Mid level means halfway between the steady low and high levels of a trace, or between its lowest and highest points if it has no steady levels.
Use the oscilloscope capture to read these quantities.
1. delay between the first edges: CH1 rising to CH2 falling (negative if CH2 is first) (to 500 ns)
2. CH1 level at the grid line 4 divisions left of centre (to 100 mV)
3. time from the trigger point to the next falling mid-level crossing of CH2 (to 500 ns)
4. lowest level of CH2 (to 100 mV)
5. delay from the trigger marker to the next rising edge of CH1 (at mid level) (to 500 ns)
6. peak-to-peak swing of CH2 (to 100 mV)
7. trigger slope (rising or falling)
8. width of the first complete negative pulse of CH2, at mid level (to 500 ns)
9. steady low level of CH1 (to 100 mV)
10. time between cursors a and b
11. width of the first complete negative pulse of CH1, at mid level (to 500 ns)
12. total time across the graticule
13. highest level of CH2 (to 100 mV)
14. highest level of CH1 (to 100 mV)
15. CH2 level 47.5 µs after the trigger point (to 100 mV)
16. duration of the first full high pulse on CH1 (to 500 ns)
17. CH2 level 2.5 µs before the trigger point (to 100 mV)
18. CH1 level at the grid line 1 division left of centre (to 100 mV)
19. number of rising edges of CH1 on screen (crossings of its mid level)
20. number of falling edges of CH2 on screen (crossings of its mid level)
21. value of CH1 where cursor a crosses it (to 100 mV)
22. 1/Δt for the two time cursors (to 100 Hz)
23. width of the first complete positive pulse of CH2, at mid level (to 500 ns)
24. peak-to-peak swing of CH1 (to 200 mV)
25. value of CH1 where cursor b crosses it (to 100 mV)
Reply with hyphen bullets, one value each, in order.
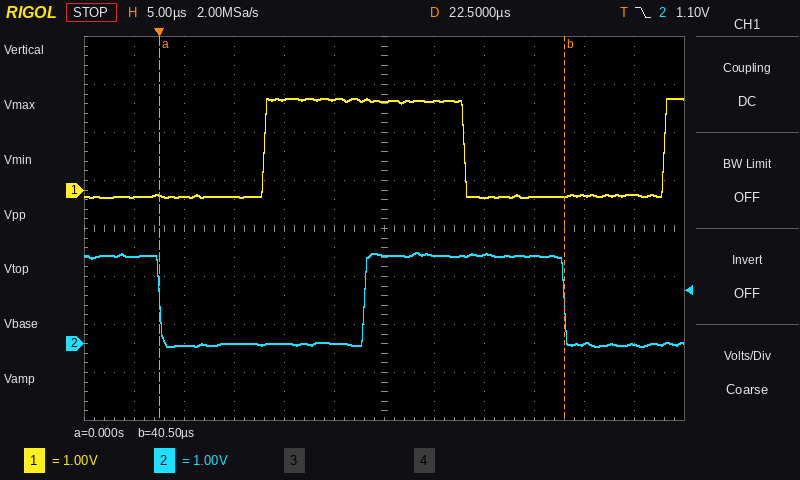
- -10.5 µs
- -100 mV
- 40.5 µs
- -100 mV
- 10.5 µs
- 2.0 V
- falling
- 20.5 µs
- -100 mV
- 40.5 µs
- 20.0 µs
- 60 µs
- 1.9 V
- 1.9 V
- 0.0 V
- 20.0 µs
- 1.8 V
- 1.9 V
- 2
- 2
- -100 mV
- 24.7 kHz
- 20.0 µs
- 2.0 V
- -100 mV
